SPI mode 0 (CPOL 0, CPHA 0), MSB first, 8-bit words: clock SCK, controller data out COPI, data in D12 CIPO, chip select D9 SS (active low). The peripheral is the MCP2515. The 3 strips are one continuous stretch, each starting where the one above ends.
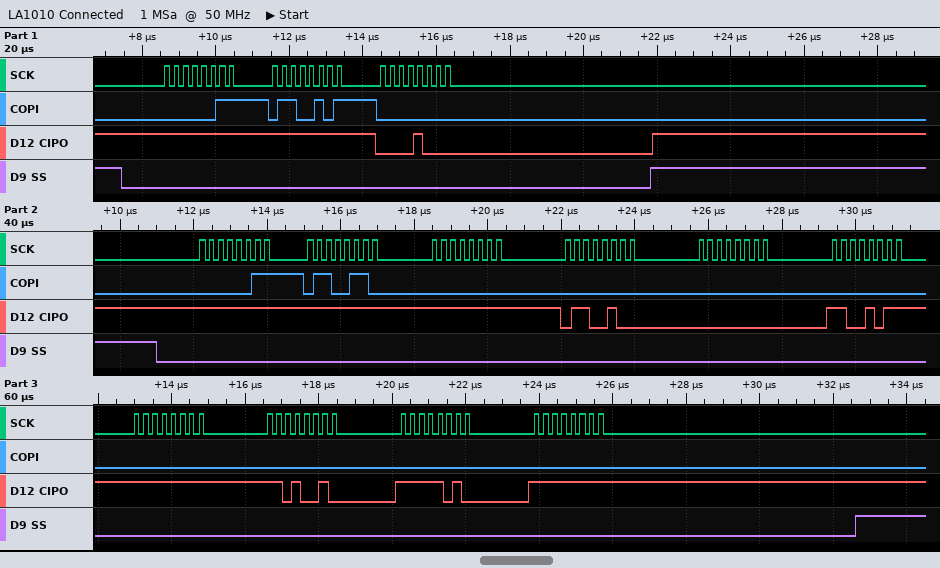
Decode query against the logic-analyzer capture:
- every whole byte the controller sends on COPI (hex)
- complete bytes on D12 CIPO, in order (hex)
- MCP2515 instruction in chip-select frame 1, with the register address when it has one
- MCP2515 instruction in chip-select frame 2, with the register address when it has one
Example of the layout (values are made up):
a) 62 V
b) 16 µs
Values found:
a) 03 65 00 03 66 00 00 00 00 00 00 00 00
b) FF FF 08 FF FF FF 64 00 CB FF D2 FA FF
c) READ 0x65
d) READ 0x66
